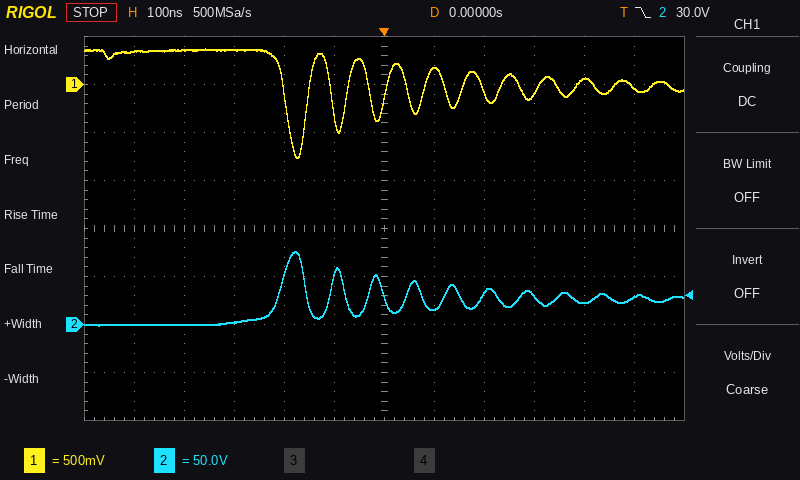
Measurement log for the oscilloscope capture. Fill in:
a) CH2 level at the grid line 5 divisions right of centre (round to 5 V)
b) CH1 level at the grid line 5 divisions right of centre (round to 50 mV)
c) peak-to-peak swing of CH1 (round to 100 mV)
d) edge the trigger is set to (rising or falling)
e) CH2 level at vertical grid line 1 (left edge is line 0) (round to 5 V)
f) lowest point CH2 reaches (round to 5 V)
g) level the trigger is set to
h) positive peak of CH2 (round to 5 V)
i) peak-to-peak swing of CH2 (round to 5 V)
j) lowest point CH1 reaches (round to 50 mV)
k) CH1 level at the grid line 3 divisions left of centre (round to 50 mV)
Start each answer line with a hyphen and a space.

- 30 V
- -50 mV
- 1.10 V
- falling
- 0 V
- 0 V
- 30.0 V
- 75 V
- 75 V
- -750 mV
- 350 mV
